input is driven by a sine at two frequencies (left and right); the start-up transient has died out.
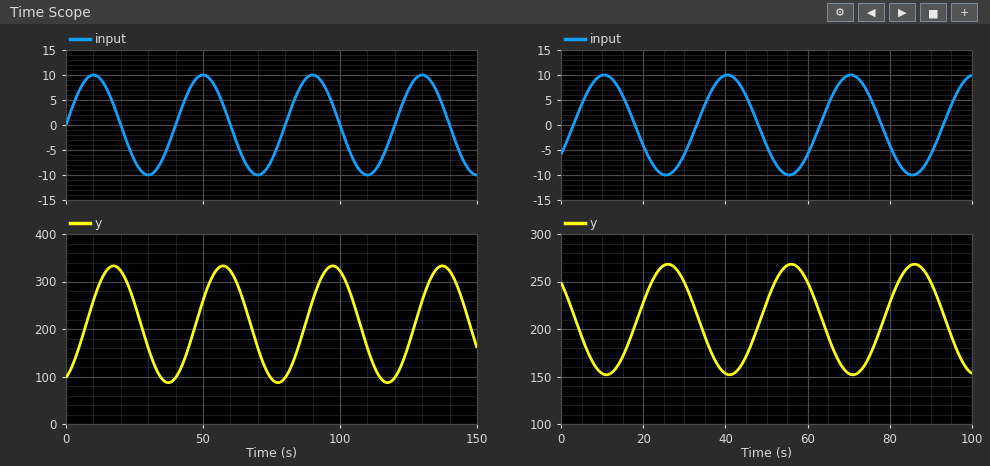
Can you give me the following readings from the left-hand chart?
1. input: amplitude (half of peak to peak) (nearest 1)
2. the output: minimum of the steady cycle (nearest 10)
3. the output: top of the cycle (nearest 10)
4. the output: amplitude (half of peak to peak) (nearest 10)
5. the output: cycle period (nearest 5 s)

10
90
330
120
40 s
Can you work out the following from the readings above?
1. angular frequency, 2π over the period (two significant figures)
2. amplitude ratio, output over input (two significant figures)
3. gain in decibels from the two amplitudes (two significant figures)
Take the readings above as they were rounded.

0.16 rad/s
12
22 dB
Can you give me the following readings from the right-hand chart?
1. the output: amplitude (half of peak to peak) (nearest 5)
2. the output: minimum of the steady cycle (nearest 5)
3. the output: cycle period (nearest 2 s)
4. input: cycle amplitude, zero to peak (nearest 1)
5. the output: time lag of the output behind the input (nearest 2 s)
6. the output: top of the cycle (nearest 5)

60
150
30 s
10
16 s
270
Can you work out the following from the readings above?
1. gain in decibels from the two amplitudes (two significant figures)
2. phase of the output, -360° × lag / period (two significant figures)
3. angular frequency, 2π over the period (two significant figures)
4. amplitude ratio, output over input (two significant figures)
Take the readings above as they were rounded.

16 dB
-190°
0.21 rad/s
6.0
